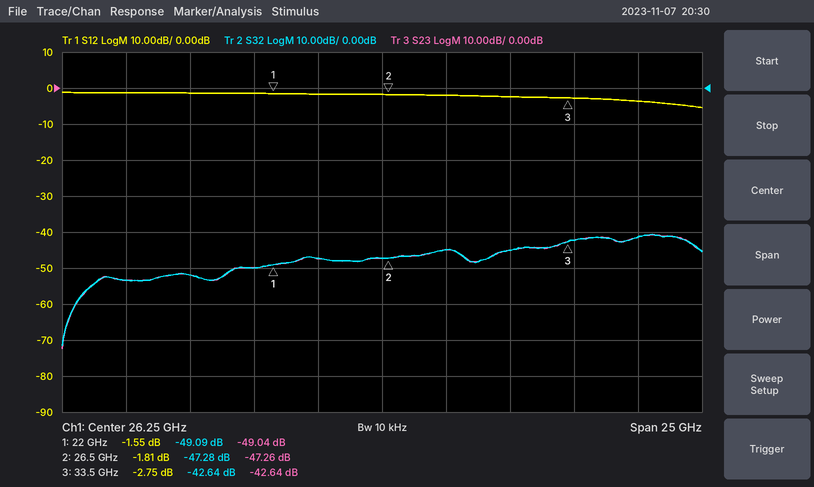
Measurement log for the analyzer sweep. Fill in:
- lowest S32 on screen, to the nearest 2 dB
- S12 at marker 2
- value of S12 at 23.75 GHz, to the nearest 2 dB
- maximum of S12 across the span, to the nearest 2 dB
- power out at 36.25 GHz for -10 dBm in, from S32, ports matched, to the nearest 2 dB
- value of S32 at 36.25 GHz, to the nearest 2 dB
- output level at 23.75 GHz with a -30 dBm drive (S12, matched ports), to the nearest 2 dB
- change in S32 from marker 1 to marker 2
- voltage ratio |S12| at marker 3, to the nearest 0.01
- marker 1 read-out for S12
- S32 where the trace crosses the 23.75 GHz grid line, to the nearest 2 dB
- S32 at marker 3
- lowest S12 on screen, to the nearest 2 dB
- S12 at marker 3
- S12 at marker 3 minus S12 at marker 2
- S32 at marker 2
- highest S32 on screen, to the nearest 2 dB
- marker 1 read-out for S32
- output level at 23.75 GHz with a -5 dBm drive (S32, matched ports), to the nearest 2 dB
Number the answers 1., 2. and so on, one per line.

1. -72 dB
2. -1.81 dB
3. -2 dB
4. -2 dB
5. -52 dBm
6. -42 dB
7. -32 dBm
8. 1.81 dB
9. 0.73
10. -1.55 dB
11. -48 dB
12. -42.64 dB
13. -6 dB
14. -2.75 dB
15. -0.94 dB
16. -47.28 dB
17. -40 dB
18. -49.09 dB
19. -52 dBm
